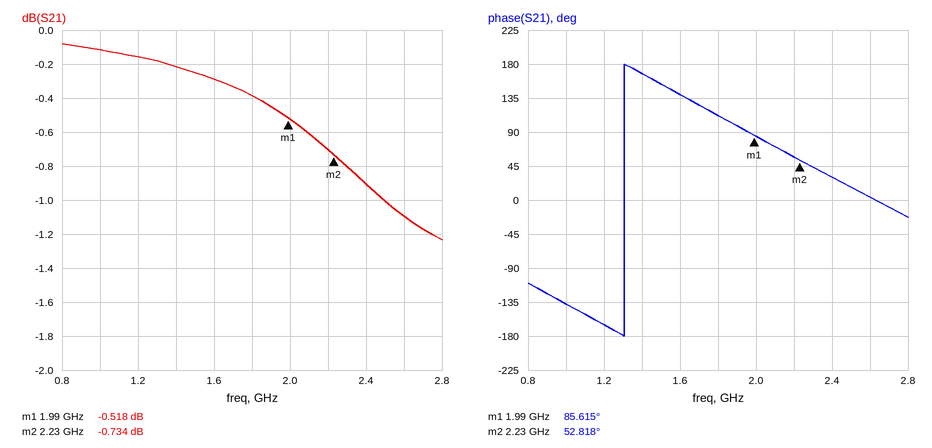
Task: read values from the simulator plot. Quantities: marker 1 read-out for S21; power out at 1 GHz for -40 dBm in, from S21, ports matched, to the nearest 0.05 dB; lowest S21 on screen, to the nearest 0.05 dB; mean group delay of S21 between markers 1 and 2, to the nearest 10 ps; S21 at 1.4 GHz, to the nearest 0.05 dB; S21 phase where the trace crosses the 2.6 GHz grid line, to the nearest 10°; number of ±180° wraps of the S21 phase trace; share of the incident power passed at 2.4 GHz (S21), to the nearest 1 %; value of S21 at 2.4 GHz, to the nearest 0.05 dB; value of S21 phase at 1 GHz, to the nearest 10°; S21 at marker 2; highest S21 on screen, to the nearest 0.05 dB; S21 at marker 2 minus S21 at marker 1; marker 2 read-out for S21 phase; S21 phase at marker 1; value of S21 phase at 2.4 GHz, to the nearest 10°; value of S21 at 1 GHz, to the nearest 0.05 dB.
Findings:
-0.518 dB
-40.10 dBm
-1.25 dB
380 ps
-0.20 dB
0°
1
81 %
-0.90 dB
-140°
-0.734 dB
-0.10 dB
-0.216 dB
52.818°
85.615°
30°
-0.10 dB
